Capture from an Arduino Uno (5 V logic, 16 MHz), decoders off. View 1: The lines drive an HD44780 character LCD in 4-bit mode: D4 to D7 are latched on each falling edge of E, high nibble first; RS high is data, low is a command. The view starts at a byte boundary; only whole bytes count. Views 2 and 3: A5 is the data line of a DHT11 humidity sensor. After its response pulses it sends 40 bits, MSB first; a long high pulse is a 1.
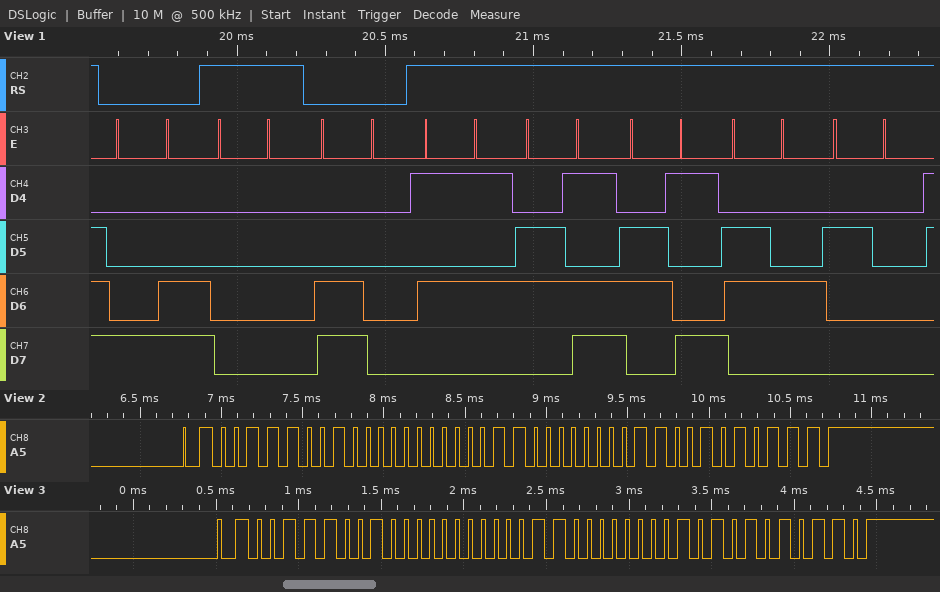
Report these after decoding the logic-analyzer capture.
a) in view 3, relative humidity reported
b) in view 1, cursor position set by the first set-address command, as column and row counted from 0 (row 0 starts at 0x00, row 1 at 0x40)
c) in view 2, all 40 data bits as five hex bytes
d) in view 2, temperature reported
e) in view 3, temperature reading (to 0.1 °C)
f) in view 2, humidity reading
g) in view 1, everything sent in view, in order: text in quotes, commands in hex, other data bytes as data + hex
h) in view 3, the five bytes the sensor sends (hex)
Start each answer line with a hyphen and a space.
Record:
- 57 %
- column 12, row 0
- 39 00 18 06 57
- 24.6 °C
- 24.5 °C
- 57 %
- 0x8C data 00 0xC0 "Umid "
- 39 00 18 05 56
